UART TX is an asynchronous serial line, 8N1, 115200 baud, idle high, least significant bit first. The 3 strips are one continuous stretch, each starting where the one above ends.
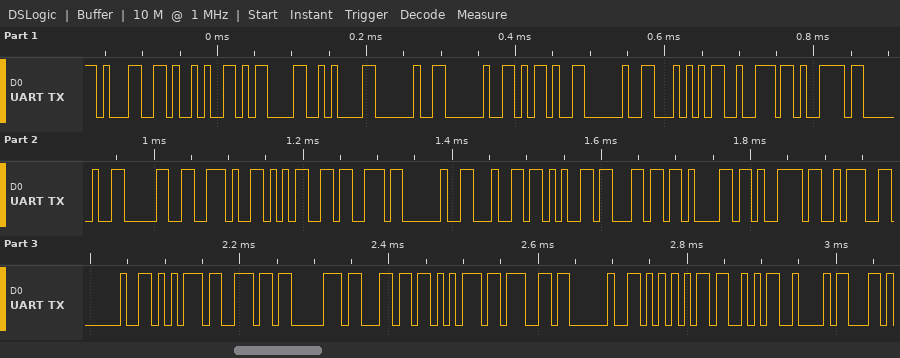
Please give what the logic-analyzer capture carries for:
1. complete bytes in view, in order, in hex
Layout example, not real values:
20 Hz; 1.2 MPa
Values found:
31 29 0D 0A 20 20 2D 20 54 72 79 20 30 2E 35 73 20 64 65 6C 61 79 3A 20 75 6E 70 6C 75 67 20 55 53 42
